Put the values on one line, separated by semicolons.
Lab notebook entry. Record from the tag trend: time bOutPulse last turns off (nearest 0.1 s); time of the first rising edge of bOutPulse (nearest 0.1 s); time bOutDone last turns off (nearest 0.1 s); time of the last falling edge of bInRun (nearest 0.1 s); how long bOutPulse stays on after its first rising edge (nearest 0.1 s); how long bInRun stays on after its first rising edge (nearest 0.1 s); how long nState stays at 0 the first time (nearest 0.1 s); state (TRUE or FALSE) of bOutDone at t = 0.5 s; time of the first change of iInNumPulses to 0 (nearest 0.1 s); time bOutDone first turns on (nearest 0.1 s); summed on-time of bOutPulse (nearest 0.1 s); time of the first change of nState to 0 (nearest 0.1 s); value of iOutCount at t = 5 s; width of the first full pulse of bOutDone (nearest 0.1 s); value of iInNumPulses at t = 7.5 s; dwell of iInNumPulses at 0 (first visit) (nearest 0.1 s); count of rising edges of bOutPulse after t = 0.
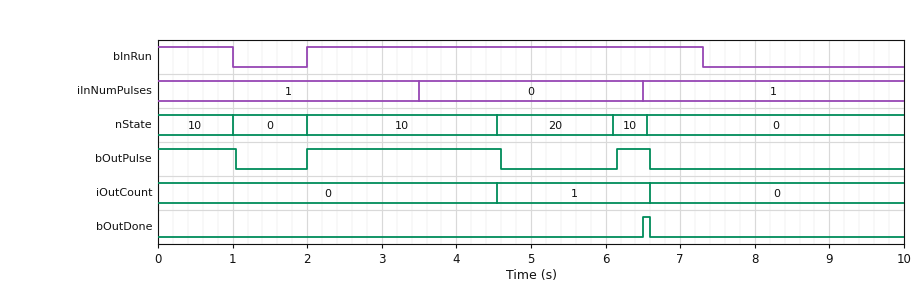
6.6 s; 2.0 s; 6.6 s; 7.3 s; 2.6 s; 5.3 s; 1.0 s; FALSE; 3.5 s; 6.5 s; 4.1 s; 1.0 s; 1; 0.1 s; 1; 3.0 s; 2
